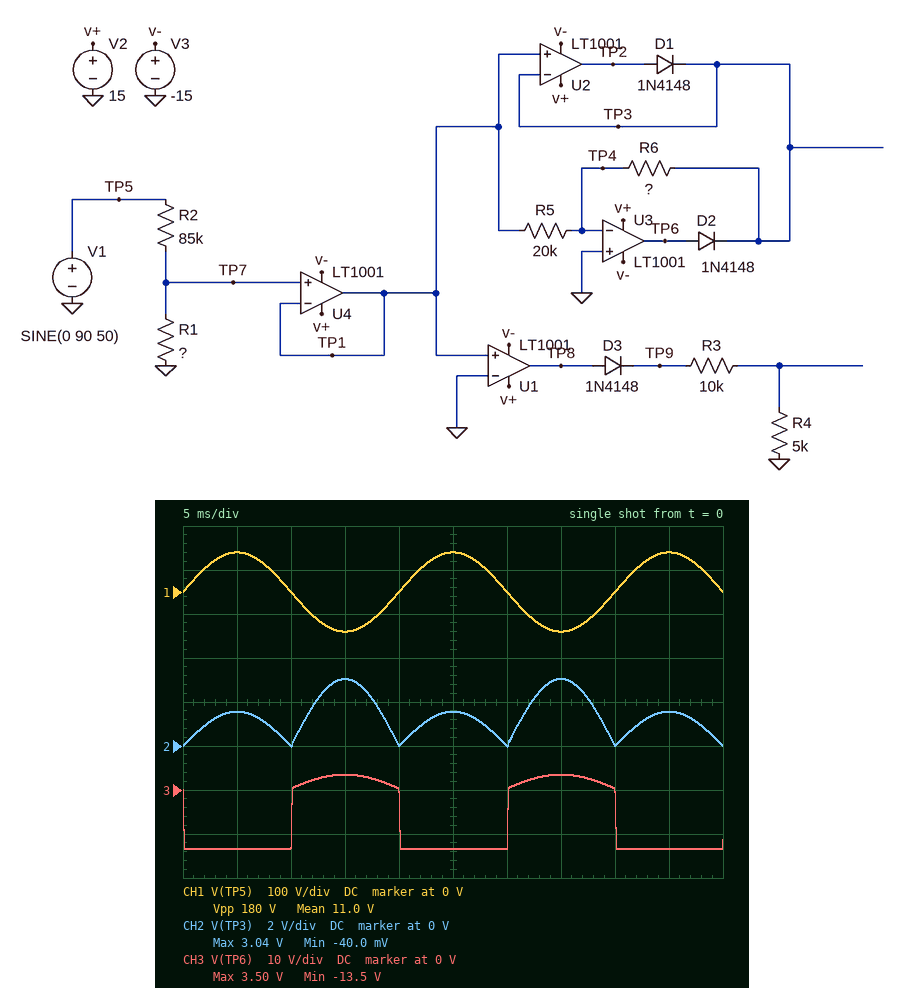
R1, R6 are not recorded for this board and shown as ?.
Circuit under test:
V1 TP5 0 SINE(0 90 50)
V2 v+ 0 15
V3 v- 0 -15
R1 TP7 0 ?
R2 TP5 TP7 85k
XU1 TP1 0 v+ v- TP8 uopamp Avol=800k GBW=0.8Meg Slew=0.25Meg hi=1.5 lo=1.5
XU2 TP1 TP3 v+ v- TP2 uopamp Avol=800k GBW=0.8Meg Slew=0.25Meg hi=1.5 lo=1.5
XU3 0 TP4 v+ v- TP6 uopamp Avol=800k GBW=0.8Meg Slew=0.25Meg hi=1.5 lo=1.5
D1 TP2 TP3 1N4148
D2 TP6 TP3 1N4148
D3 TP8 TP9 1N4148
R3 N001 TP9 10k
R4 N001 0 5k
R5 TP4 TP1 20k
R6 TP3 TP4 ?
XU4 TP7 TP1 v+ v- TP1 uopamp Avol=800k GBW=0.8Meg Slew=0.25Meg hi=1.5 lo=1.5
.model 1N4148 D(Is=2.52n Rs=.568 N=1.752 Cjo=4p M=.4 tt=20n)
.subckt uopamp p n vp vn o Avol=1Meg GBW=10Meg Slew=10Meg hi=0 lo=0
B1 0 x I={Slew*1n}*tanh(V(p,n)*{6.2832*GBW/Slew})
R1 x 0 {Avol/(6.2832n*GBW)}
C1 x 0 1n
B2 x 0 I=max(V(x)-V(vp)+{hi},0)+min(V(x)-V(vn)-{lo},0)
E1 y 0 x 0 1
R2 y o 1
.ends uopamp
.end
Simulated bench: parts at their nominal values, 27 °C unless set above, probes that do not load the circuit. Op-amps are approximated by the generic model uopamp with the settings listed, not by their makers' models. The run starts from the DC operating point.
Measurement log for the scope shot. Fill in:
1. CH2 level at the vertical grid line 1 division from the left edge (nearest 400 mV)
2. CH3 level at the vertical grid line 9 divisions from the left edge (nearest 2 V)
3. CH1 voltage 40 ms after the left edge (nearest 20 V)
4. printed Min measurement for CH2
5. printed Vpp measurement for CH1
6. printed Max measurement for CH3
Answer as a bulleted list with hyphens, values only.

- 1.6 V
- -14 V
- 0 V
- -40.0 mV
- 180 V
- 3.50 V
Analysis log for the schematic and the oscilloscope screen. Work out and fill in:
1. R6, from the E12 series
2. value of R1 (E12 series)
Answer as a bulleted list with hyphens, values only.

- 39 kΩ
- 1.5 kΩ
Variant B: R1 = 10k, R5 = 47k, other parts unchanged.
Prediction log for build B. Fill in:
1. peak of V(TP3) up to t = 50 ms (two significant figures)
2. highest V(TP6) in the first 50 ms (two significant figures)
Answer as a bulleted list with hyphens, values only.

- 9.5 V
- 8.4 V
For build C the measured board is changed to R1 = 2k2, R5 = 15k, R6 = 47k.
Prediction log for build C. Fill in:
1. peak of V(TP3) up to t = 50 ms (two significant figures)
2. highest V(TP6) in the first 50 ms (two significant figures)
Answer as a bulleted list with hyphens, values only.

- 7.1 V
- 7.6 V
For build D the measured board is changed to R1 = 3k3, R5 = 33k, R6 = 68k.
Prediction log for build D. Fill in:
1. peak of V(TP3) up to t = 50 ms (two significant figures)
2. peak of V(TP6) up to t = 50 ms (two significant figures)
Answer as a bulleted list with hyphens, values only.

- 6.9 V
- 7.4 V
